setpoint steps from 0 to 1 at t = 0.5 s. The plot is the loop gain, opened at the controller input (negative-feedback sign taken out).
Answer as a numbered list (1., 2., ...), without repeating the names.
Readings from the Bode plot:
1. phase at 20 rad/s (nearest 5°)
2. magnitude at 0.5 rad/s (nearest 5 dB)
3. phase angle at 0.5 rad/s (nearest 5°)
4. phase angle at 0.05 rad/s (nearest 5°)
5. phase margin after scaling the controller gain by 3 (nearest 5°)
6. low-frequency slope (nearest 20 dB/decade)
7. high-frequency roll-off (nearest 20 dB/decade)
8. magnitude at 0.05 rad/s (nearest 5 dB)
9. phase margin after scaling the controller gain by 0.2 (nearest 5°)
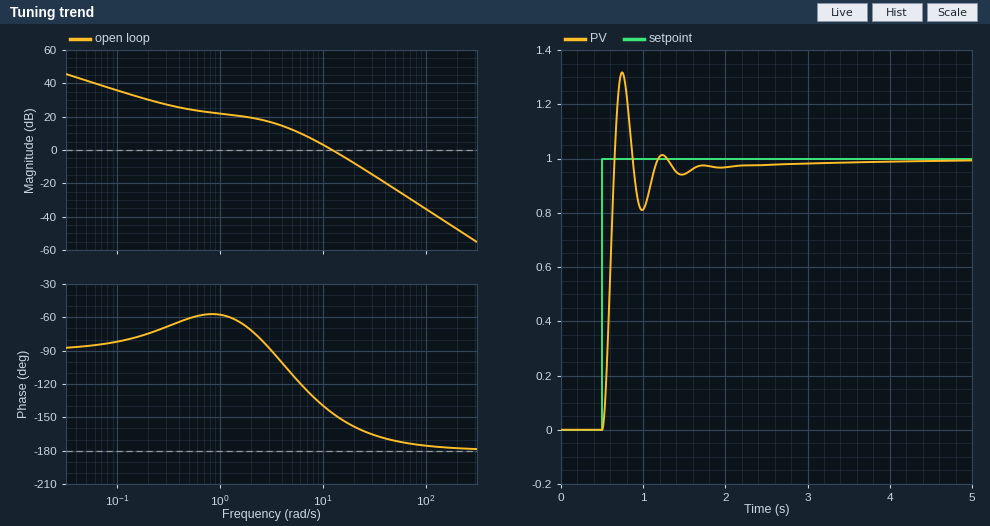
1. -160°
2. 25 dB
3. -60°
4. -85°
5. 20°
6. -20 dB/decade
7. -40 dB/decade
8. 40 dB
9. 75°
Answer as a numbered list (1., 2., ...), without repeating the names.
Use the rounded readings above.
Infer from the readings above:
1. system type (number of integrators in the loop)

1. 1
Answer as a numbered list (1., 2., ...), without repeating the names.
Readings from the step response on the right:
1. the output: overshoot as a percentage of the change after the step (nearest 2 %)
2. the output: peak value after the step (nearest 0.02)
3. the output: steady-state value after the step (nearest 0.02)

1. 32 %
2. 1.32
3. 1.00
